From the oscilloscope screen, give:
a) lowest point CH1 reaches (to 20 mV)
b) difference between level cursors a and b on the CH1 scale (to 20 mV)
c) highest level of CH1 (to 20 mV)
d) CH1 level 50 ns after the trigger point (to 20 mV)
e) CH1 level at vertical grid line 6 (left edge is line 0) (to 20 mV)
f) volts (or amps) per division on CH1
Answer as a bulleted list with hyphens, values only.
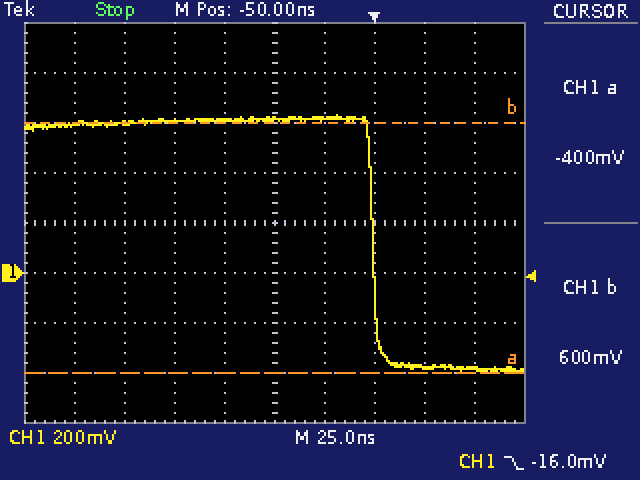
- -400 mV
- 1.00 V
- 640 mV
- -380 mV
- 620 mV
- 200 mV
